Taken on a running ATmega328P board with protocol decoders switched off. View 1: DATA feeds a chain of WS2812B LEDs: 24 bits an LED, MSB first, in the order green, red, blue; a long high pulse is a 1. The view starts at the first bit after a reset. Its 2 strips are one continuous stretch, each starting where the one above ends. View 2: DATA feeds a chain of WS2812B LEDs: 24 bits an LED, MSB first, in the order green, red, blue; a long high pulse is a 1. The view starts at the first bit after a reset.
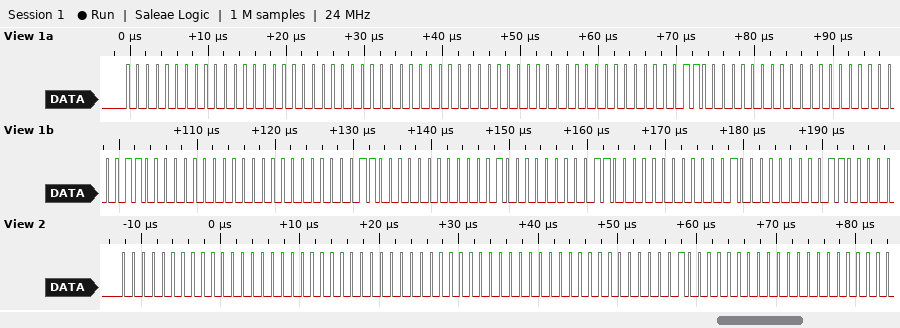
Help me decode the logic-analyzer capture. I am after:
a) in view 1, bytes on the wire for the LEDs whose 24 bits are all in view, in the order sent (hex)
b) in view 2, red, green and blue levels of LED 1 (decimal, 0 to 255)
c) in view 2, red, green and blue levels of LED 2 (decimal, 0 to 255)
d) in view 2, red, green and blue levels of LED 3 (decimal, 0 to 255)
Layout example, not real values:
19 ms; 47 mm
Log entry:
00 00 00 00 00 00 00 60 00 00 60 00 00 60 01 00 60 01; 0, 0, 0; 0, 0, 0; 128, 0, 0
